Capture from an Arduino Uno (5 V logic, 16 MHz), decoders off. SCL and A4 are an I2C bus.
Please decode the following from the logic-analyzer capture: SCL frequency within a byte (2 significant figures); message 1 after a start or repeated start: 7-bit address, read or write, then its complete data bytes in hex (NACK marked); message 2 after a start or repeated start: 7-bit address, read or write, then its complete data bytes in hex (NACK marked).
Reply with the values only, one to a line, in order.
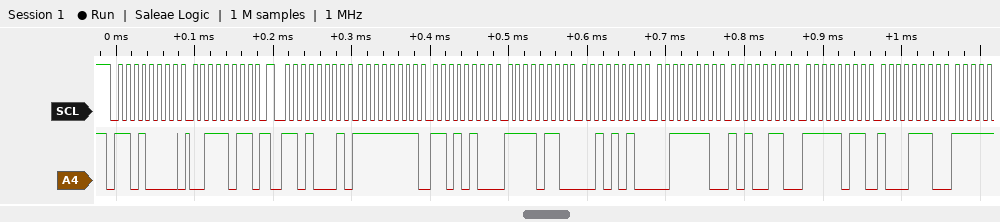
100 kHz
0x68 write: 3B
0x68 read: FF D4 F6 2A 3E A6 FB 8E
